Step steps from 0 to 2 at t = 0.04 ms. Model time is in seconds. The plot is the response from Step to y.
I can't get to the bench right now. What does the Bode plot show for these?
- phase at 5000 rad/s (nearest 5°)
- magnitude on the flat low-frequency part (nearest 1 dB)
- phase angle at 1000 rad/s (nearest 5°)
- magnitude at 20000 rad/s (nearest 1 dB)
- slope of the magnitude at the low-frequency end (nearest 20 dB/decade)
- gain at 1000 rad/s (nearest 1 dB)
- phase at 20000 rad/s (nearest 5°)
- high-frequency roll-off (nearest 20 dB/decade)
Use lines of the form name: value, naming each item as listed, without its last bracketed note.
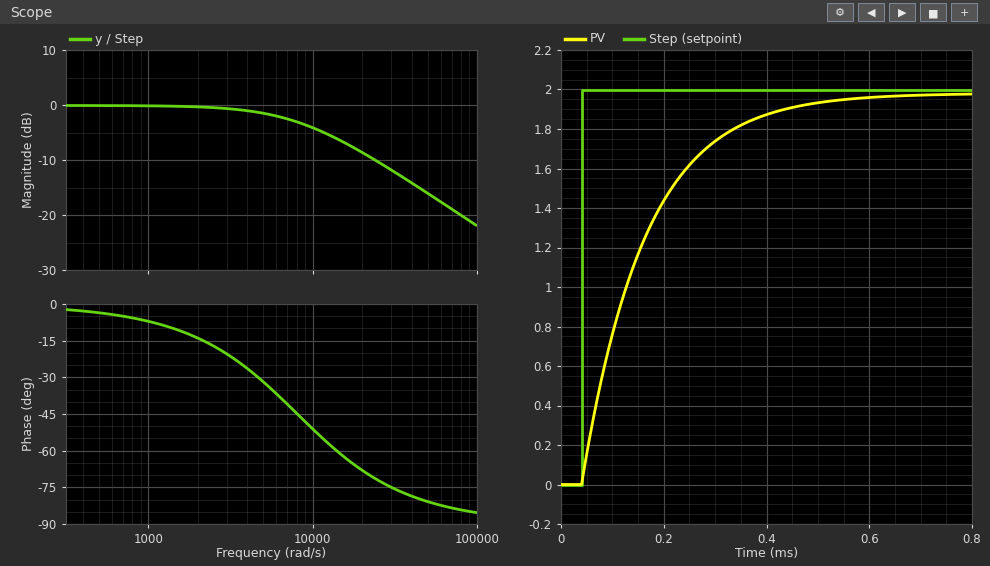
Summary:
phase at 5000 rad/s: -30°
magnitude on the flat low-frequency part: 0 dB
phase angle at 1000 rad/s: -5°
magnitude at 20000 rad/s: -9 dB
slope of the magnitude at the low-frequency end: 0 dB/decade
gain at 1000 rad/s: 0 dB
phase at 20000 rad/s: -70°
high-frequency roll-off: -20 dB/decade
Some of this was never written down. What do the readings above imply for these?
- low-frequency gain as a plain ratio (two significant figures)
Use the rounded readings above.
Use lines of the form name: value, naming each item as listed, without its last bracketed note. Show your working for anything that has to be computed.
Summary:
low-frequency gain as a plain ratio: 10^(0 / 20) = 1.0
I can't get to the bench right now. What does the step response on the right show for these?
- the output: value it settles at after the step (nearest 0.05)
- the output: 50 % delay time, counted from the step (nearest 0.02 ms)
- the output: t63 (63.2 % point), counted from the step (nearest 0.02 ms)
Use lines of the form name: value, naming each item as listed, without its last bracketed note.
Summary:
the output: value it settles at after the step: 2.00
the output: 50 % delay time, counted from the step: 0.08 ms
the output: t63 (63.2 % point), counted from the step: 0.12 ms
